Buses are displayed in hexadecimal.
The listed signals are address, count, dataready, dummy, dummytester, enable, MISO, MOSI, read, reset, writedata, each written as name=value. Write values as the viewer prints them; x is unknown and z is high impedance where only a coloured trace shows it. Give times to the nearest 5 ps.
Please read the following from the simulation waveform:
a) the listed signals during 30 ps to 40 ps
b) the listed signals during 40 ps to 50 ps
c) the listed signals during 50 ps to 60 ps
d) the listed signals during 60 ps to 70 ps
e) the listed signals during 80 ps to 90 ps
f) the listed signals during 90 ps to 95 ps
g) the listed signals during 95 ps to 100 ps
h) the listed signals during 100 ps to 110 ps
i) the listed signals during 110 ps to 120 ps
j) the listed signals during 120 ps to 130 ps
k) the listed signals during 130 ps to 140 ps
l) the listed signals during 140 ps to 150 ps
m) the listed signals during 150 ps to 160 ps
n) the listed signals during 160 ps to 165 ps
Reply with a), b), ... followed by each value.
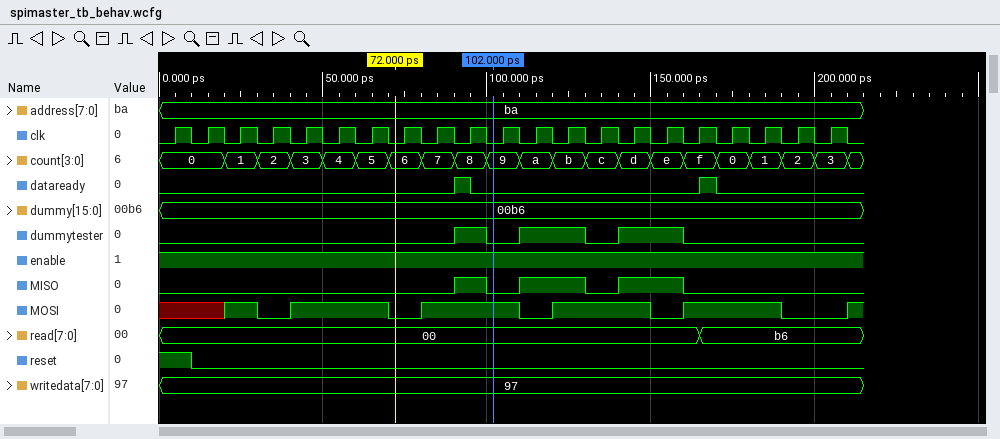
a) address=ba, count=2, dataready=0, dummy=00b6, dummytester=0, enable=1, MISO=0, MOSI=0, read=00, reset=0, writedata=97
b) address=ba, count=3, dataready=0, dummy=00b6, dummytester=0, enable=1, MISO=0, MOSI=1, read=00, reset=0, writedata=97
c) address=ba, count=4, dataready=0, dummy=00b6, dummytester=0, enable=1, MISO=0, MOSI=1, read=00, reset=0, writedata=97
d) address=ba, count=5, dataready=0, dummy=00b6, dummytester=0, enable=1, MISO=0, MOSI=1, read=00, reset=0, writedata=97
e) address=ba, count=7, dataready=0, dummy=00b6, dummytester=0, enable=1, MISO=0, MOSI=1, read=00, reset=0, writedata=97
f) address=ba, count=8, dataready=1, dummy=00b6, dummytester=1, enable=1, MISO=1, MOSI=1, read=00, reset=0, writedata=97
g) address=ba, count=8, dataready=0, dummy=00b6, dummytester=1, enable=1, MISO=1, MOSI=1, read=00, reset=0, writedata=97
h) address=ba, count=9, dataready=0, dummy=00b6, dummytester=0, enable=1, MISO=0, MOSI=1, read=00, reset=0, writedata=97
i) address=ba, count=a, dataready=0, dummy=00b6, dummytester=1, enable=1, MISO=1, MOSI=0, read=00, reset=0, writedata=97
j) address=ba, count=b, dataready=0, dummy=00b6, dummytester=1, enable=1, MISO=1, MOSI=1, read=00, reset=0, writedata=97
k) address=ba, count=c, dataready=0, dummy=00b6, dummytester=0, enable=1, MISO=0, MOSI=1, read=00, reset=0, writedata=97
l) address=ba, count=d, dataready=0, dummy=00b6, dummytester=1, enable=1, MISO=1, MOSI=1, read=00, reset=0, writedata=97
m) address=ba, count=e, dataready=0, dummy=00b6, dummytester=1, enable=1, MISO=1, MOSI=0, read=00, reset=0, writedata=97
n) address=ba, count=f, dataready=0, dummy=00b6, dummytester=0, enable=1, MISO=0, MOSI=1, read=00, reset=0, writedata=97
